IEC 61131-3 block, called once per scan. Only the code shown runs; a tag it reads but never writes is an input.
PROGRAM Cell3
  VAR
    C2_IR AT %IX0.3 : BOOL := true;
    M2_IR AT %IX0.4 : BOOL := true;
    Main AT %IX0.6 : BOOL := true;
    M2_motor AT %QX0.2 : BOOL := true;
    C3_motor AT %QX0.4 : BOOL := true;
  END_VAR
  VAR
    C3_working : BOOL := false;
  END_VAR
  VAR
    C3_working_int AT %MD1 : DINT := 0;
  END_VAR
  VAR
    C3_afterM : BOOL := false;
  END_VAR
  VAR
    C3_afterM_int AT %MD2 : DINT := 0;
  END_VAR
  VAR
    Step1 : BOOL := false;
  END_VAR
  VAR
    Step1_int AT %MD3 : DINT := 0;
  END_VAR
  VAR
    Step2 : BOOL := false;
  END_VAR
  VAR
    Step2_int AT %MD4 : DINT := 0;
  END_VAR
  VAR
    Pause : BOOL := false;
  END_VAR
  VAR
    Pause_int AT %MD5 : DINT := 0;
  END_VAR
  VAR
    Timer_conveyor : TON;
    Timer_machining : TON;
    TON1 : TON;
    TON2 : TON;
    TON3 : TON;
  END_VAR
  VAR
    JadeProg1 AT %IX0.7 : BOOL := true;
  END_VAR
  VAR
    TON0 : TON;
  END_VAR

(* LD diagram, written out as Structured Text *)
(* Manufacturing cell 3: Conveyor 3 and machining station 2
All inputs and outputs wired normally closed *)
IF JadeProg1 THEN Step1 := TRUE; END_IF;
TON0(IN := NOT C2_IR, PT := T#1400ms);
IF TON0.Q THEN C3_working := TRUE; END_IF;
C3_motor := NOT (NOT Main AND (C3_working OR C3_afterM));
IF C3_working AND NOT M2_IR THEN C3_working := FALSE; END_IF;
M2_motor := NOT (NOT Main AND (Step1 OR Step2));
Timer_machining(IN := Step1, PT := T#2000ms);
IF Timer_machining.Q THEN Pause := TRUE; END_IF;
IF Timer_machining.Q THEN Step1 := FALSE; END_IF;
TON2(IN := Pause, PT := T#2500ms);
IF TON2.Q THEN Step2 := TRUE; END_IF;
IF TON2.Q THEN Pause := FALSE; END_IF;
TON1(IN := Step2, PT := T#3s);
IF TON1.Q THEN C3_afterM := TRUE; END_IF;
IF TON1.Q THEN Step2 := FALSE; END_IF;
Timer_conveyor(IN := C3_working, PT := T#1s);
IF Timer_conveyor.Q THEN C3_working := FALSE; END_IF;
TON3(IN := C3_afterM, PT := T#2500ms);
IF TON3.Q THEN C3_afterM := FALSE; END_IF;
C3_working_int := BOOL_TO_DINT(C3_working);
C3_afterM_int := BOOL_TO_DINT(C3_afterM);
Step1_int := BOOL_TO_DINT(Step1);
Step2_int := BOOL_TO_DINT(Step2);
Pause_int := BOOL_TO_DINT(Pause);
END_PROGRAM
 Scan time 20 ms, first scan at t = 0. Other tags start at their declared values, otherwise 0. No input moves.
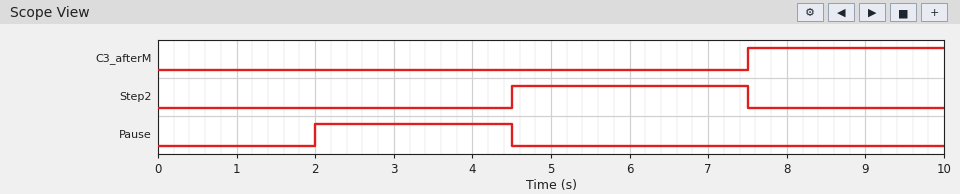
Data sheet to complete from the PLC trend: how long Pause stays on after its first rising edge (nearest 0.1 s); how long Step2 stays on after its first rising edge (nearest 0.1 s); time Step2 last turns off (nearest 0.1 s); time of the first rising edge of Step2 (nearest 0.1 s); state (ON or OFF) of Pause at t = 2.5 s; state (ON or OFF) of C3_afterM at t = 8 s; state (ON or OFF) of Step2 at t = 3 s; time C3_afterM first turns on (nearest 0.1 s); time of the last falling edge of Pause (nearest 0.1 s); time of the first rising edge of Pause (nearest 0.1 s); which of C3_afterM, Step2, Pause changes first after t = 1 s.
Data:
2.5 s
3.0 s
7.5 s
4.5 s
ON
ON
OFF
7.5 s
4.5 s
2.0 s
Pause
